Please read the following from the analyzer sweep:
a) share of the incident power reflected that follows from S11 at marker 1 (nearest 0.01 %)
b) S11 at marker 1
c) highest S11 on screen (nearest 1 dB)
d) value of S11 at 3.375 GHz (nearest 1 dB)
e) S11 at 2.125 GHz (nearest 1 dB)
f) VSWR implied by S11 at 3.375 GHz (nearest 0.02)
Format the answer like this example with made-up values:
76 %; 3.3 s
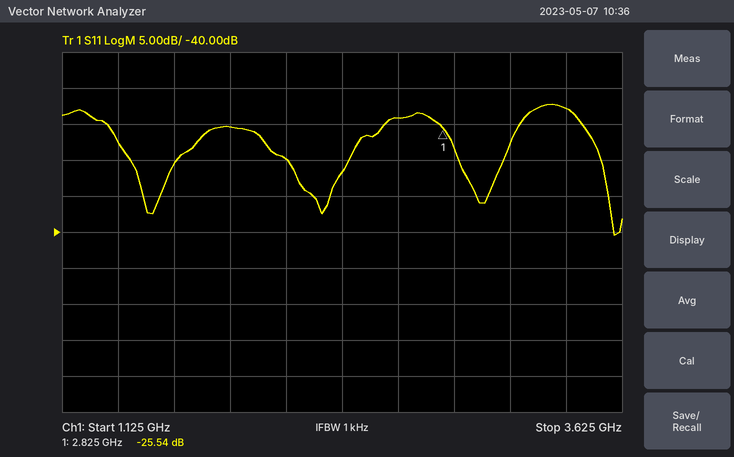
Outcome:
0.28 %; -25.54 dB; -22 dB; -23 dB; -30 dB; 1.16
